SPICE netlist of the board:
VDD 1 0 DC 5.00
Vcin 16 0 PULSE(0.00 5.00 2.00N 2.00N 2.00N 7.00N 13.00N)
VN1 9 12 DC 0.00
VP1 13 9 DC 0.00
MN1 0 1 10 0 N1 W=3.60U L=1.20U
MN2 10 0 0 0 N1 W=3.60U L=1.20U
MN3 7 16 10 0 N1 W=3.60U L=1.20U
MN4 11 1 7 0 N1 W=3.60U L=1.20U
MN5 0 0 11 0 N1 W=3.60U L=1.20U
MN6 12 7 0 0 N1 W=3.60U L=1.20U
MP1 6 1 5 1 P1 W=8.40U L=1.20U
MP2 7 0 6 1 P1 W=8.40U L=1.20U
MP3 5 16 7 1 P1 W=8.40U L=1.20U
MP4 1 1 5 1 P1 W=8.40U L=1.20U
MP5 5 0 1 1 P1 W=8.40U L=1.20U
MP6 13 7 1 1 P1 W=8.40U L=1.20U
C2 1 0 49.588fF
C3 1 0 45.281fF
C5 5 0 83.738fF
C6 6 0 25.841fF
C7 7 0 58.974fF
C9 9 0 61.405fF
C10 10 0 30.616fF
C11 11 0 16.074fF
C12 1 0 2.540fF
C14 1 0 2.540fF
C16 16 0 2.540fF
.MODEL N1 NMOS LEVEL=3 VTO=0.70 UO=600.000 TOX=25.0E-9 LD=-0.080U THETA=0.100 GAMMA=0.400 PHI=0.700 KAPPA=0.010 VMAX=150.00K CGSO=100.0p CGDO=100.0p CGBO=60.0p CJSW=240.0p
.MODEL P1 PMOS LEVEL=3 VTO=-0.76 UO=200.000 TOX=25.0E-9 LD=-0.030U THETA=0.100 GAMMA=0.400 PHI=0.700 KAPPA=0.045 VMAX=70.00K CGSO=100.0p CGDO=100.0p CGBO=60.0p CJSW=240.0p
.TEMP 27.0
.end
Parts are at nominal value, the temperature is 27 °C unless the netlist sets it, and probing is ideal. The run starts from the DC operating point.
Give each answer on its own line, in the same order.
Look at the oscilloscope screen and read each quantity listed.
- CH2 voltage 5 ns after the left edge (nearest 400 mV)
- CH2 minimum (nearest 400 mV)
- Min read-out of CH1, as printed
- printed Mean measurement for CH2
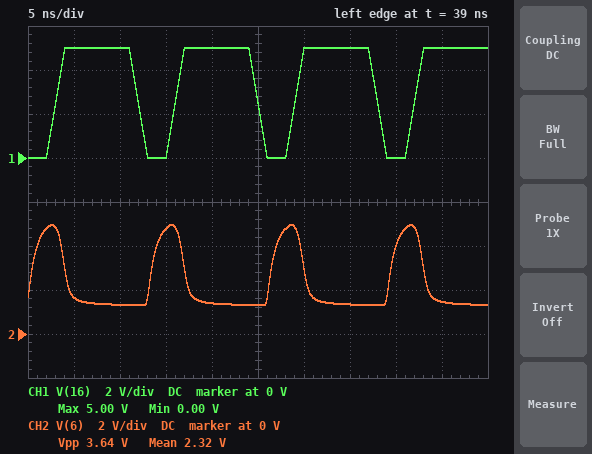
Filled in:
1.6 V
1.2 V
0.00 V
2.32 V
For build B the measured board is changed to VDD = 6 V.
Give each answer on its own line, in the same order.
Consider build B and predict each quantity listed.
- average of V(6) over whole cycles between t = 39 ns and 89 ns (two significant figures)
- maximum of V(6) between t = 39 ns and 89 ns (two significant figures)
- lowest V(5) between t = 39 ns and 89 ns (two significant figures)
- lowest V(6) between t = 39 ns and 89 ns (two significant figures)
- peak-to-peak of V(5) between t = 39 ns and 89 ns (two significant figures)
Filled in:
2.8 V
6.0 V
4.9 V
1.4 V
1.1 V
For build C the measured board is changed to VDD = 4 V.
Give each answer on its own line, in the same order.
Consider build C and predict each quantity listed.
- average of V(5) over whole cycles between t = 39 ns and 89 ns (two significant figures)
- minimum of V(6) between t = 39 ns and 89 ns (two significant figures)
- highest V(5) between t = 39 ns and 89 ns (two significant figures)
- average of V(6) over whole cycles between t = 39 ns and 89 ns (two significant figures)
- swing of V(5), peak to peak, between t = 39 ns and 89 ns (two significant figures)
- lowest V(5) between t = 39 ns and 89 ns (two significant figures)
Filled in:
3.9 V
1.2 V
4.0 V
1.8 V
770 mV
3.3 V
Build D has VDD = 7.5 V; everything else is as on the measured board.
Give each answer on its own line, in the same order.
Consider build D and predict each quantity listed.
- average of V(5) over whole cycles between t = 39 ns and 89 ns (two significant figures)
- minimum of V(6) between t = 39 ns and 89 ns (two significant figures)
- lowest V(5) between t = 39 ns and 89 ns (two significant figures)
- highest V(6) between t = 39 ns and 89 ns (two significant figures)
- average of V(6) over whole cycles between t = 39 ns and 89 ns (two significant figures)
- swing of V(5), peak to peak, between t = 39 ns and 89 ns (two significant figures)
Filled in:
7.2 V
1.5 V
6.3 V
7.5 V
3.7 V
1.2 V
